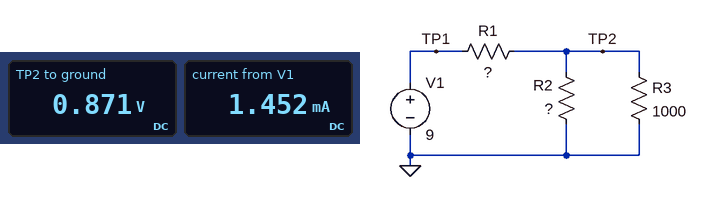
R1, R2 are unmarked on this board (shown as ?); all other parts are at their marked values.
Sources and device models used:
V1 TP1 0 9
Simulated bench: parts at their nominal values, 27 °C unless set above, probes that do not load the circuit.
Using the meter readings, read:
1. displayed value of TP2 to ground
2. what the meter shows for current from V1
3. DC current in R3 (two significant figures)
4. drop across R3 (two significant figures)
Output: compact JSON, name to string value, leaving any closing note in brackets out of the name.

{"displayed value of TP2 to ground": "0.871 V", "what the meter shows for current from V1": "1.452 mA", "DC current in R3": "870 µA", "drop across R3": "870 mV"}
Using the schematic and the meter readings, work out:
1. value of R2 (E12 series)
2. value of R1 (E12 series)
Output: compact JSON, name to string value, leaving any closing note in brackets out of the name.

{"value of R2": "1.5 kΩ", "value of R1": "5.6 kΩ"}
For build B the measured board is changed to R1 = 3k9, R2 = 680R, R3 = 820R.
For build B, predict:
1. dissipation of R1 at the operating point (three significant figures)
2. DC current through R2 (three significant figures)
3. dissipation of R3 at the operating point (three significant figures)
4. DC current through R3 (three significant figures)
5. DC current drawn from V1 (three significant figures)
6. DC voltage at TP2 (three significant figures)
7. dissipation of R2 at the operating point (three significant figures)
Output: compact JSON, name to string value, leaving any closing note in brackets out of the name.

{"dissipation of R1 at the operating point": "17.3 mW", "DC current through R2": "1.15 mA", "dissipation of R3 at the operating point": "748 µW", "DC current through R3": "955 µA", "DC current drawn from V1": "2.11 mA", "DC voltage at TP2": "783 mV", "dissipation of R2 at the operating point": "902 µW"}
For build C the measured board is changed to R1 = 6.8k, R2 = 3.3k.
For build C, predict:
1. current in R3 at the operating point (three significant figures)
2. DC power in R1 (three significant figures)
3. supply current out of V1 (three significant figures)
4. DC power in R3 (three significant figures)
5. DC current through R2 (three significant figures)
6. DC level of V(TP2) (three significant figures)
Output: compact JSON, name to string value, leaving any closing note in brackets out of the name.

{"current in R3 at the operating point": "913 µA", "DC power in R1": "9.62 mW", "supply current out of V1": "1.19 mA", "DC power in R3": "833 µW", "DC current through R2": "277 µA", "DC level of V(TP2)": "913 mV"}
